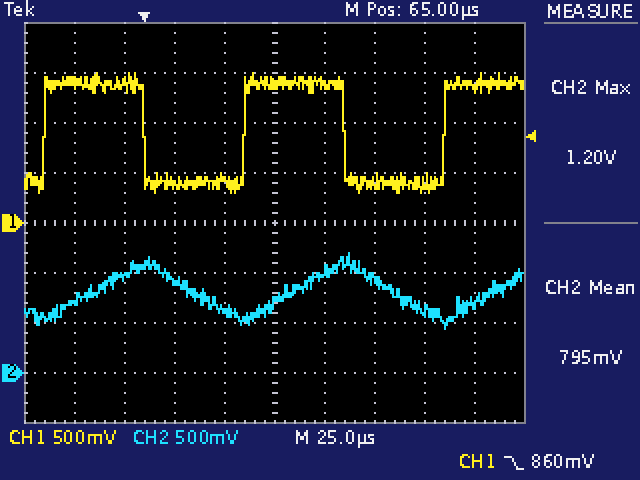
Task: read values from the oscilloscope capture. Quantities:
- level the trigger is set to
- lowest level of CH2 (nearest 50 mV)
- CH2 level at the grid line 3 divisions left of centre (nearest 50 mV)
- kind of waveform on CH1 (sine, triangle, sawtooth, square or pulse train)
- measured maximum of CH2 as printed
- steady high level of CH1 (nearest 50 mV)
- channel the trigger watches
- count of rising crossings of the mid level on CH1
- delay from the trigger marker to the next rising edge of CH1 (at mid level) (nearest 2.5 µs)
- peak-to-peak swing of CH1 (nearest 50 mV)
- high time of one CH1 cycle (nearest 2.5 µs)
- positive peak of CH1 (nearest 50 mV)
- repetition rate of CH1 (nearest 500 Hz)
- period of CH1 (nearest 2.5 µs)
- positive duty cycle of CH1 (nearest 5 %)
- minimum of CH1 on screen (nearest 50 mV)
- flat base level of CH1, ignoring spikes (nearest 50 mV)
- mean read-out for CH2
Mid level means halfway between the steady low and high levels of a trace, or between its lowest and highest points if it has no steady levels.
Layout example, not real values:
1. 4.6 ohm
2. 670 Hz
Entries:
1. 860 mV
2. 450 mV
3. 950 mV
4. square
5. 1.20 V
6. 1.40 V
7. CH1
8. 3
9. 50.0 µs
10. 1.20 V
11. 50.0 µs
12. 1.50 V
13. 10.0 kHz
14. 100.0 µs
15. 50 %
16. 300 mV
17. 400 mV
18. 795 mV
